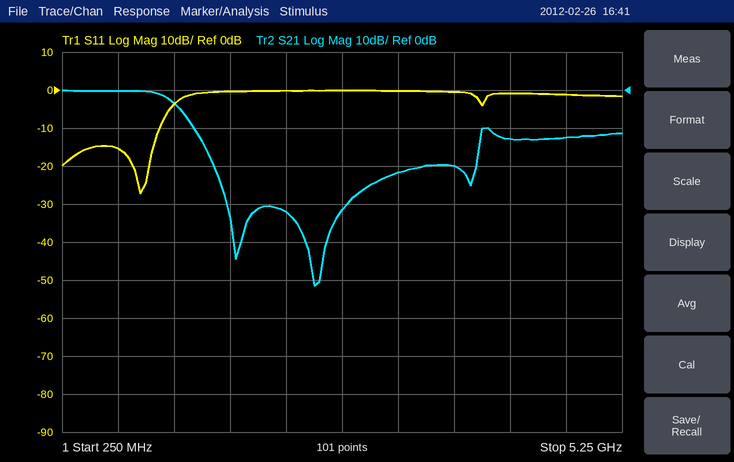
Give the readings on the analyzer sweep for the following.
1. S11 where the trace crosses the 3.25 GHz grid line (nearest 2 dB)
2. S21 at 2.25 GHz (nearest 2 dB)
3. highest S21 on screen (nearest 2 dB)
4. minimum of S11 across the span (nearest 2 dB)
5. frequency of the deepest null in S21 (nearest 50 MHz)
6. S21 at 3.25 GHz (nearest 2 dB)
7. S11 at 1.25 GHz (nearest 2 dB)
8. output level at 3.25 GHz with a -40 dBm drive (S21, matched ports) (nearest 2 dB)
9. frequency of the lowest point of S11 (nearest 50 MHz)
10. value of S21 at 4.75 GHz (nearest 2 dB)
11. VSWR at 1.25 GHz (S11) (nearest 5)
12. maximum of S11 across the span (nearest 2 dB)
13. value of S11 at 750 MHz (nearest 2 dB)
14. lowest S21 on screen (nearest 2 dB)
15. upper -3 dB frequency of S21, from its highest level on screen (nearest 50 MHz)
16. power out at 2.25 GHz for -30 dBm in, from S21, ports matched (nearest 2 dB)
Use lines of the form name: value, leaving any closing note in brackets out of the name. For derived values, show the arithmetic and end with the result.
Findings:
S11 where the trace crosses the 3.25 GHz grid line: 0 dB
S21 at 2.25 GHz: -32 dB
highest S21 on screen: 0 dB
minimum of S11 across the span: -28 dB
frequency of the deepest null in S21: 2.50 GHz
S21 at 3.25 GHz: -22 dB
S11 at 1.25 GHz: -4 dB
output level at 3.25 GHz with a -40 dBm drive (S21, matched ports): -40 dBm + (-22 dB) = -62 dBm
frequency of the lowest point of S11: 950 MHz
value of S21 at 4.75 GHz: -12 dB
VSWR at 1.25 GHz (S11): |Γ| = 10^(-4/20) = 0.6310; VSWR = (1 + 0.6310)/(1 − 0.6310) ≈ 4.42, so 5 to the nearest 5
maximum of S11 across the span: 0 dB
value of S11 at 750 MHz: -16 dB
lowest S21 on screen: -52 dB
upper -3 dB frequency of S21, from its highest level on screen: 1.25 GHz
power out at 2.25 GHz for -30 dBm in, from S21, ports matched: -30 dBm + (-32 dB) = -62 dBm
